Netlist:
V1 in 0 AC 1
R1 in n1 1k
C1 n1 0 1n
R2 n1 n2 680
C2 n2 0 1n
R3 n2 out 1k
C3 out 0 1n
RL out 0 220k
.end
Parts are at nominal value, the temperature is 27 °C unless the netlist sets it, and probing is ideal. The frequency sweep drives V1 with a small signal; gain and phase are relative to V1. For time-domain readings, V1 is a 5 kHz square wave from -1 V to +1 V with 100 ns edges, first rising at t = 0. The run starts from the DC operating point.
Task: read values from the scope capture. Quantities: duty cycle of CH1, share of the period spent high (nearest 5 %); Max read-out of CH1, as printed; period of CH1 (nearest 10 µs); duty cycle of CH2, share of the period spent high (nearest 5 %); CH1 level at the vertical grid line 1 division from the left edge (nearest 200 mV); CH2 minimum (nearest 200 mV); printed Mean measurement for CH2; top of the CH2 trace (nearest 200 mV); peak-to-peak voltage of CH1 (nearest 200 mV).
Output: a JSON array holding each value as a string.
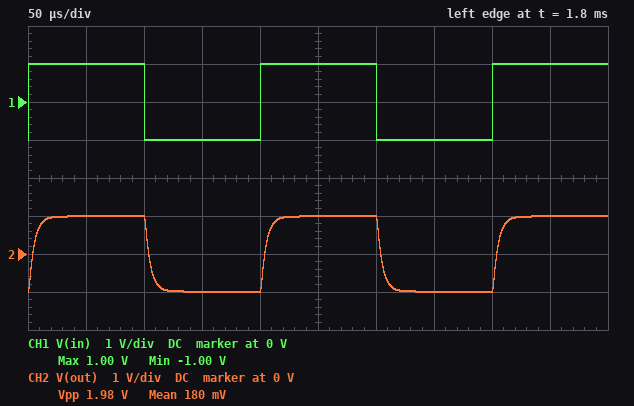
["50 %", "1.00 V", "200 µs", "50 %", "1.0 V", "-1.0 V", "180 mV", "1.0 V", "2.0 V"]
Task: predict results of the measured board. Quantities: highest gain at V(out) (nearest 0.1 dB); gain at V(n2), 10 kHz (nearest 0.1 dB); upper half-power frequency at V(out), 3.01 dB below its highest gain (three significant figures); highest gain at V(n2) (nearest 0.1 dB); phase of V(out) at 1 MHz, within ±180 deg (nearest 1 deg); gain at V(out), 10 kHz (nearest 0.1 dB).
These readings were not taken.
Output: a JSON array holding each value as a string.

["-0.1 dB", "-0.4 dB", "35.0 kHz", "-0.1 dB", "140 deg", "-0.4 dB"]
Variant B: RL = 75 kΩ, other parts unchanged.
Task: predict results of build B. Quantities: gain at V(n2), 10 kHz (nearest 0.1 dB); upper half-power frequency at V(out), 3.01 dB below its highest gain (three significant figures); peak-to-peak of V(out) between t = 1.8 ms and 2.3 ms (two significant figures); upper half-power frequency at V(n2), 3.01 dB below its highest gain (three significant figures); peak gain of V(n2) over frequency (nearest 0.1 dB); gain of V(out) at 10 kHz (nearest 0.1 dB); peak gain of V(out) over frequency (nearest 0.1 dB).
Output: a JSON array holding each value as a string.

["-0.5 dB", "35.7 kHz", "1.9 V", "37.6 kHz", "-0.2 dB", "-0.6 dB", "-0.3 dB"]
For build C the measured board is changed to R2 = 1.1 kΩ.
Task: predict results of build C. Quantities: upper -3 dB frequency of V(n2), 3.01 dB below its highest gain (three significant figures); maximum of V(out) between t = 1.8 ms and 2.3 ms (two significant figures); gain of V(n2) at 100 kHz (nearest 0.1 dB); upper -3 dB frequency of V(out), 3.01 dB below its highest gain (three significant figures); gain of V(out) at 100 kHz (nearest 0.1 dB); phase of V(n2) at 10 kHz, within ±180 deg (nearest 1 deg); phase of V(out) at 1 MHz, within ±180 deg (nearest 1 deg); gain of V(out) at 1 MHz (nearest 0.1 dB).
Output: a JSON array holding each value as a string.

["31.4 kHz", "990 mV", "-10.1 dB", "30.3 kHz", "-11.6 dB", "-18 deg", "132 deg", "-49.9 dB"]
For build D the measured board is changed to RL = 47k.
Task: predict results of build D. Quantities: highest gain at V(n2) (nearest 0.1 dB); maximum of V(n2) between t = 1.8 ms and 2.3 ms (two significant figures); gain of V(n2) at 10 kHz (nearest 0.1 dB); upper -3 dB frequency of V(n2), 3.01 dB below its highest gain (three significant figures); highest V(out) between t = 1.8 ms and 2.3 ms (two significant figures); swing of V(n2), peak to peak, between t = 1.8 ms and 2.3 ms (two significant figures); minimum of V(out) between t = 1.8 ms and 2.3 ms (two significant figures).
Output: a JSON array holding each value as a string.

["-0.3 dB", "970 mV", "-0.6 dB", "38.3 kHz", "950 mV", "1.9 V", "-950 mV"]
